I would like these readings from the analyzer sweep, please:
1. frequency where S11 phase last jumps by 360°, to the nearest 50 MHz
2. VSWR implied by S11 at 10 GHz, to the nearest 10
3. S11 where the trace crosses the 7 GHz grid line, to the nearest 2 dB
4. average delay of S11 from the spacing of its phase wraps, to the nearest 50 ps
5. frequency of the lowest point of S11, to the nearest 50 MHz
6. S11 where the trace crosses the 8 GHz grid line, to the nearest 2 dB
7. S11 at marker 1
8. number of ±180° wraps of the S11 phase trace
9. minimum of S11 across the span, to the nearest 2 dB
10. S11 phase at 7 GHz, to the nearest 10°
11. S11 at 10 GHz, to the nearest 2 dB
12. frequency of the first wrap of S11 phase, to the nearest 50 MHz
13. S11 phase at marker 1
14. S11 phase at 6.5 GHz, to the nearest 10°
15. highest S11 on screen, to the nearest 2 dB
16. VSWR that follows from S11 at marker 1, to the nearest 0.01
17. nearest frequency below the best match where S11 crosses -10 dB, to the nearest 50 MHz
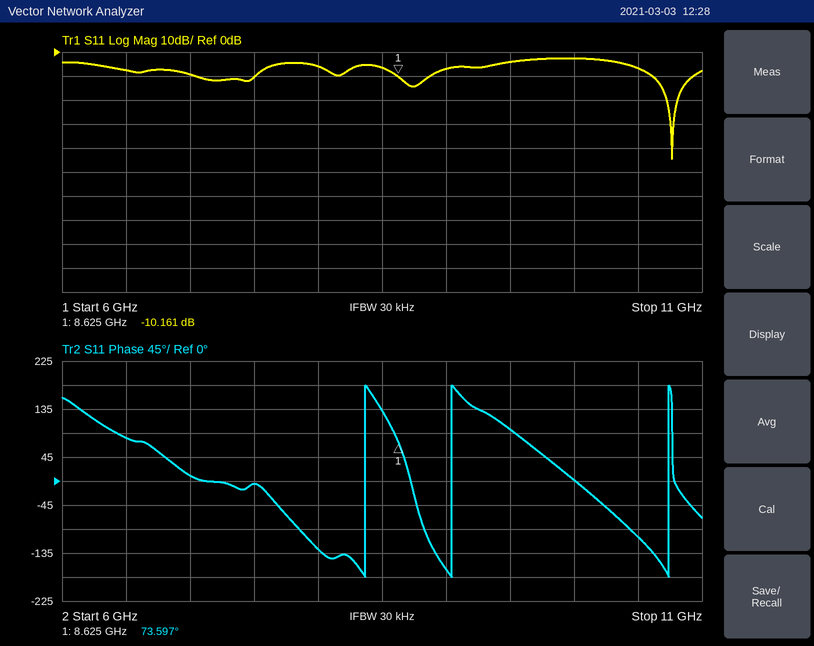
10.75 GHz
10
-10 dB
850 ps
10.75 GHz
-6 dB
-10.161 dB
3
-44 dB
10°
-2 dB
8.35 GHz
73.597°
80°
-2 dB
1.90
10.60 GHz
